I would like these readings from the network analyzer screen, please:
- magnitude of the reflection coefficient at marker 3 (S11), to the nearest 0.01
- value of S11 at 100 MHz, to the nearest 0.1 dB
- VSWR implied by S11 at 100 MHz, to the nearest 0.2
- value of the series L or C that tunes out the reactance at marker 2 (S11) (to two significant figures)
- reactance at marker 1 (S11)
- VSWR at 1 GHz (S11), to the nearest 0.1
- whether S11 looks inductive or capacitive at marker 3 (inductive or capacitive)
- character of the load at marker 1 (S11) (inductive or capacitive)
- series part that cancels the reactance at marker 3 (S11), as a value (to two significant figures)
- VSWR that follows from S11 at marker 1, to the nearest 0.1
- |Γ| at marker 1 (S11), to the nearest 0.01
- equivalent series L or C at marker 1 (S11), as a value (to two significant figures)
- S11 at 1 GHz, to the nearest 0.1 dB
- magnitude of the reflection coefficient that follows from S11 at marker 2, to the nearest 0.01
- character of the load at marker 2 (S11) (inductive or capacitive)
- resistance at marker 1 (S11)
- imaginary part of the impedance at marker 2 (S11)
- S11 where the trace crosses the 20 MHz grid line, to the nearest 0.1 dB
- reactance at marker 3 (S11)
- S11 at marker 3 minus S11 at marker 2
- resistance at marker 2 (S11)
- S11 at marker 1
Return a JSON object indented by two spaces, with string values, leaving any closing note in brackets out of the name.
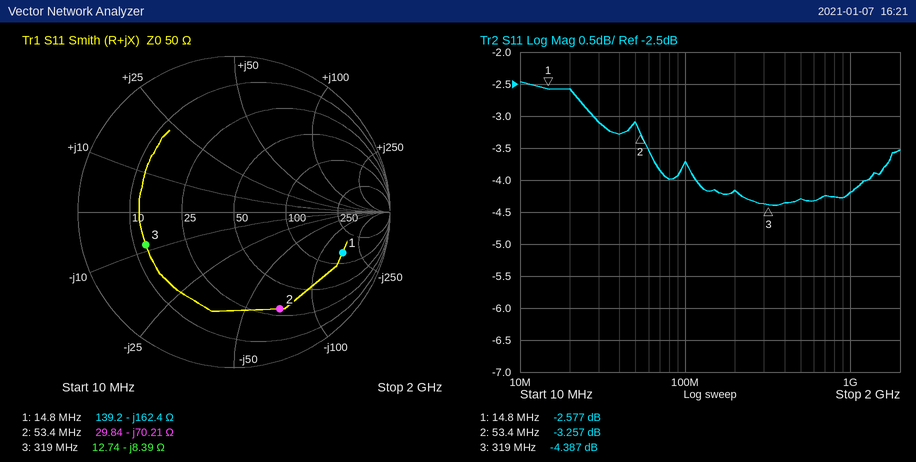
{
  "magnitude of the reflection coefficient at marker 3 (S11), to the nearest 0.01": "0.60",
  "value of S11 at 100 MHz, to the nearest 0.1 dB": "-3.7 dB",
  "VSWR implied by S11 at 100 MHz, to the nearest 0.2": "4.8",
  "value of the series L or C that tunes out the reactance at marker 2 (S11)": "210 nH",
  "reactance at marker 1": "-162.4 Ω",
  "VSWR at 1 GHz (S11), to the nearest 0.1": "4.2",
  "whether S11 looks inductive or capacitive at marker 3": "capacitive",
  "character of the load at marker 1 (S11)": "capacitive",
  "series part that cancels the reactance at marker 3 (S11), as a value": "4.2 nH",
  "VSWR that follows from S11 at marker 1, to the nearest 0.1": "6.8",
  "|Γ| at marker 1 (S11), to the nearest 0.01": "0.74",
  "equivalent series L or C at marker 1 (S11), as a value": "66 pF",
  "S11 at 1 GHz, to the nearest 0.1 dB": "-4.2 dB",
  "magnitude of the reflection coefficient that follows from S11 at marker 2, to the nearest 0.01": "0.69",
  "character of the load at marker 2 (S11)": "capacitive",
  "resistance at marker 1": "139.2 Ω",
  "imaginary part of the impedance at marker 2": "-70.21 Ω",
  "S11 where the trace crosses the 20 MHz grid line, to the nearest 0.1 dB": "-2.6 dB",
  "reactance at marker 3": "-8.39 Ω",
  "S11 at marker 3 minus S11 at marker 2": "-1.130 dB",
  "resistance at marker 2": "29.84 Ω",
  "S11 at marker 1": "-2.577 dB"
}
